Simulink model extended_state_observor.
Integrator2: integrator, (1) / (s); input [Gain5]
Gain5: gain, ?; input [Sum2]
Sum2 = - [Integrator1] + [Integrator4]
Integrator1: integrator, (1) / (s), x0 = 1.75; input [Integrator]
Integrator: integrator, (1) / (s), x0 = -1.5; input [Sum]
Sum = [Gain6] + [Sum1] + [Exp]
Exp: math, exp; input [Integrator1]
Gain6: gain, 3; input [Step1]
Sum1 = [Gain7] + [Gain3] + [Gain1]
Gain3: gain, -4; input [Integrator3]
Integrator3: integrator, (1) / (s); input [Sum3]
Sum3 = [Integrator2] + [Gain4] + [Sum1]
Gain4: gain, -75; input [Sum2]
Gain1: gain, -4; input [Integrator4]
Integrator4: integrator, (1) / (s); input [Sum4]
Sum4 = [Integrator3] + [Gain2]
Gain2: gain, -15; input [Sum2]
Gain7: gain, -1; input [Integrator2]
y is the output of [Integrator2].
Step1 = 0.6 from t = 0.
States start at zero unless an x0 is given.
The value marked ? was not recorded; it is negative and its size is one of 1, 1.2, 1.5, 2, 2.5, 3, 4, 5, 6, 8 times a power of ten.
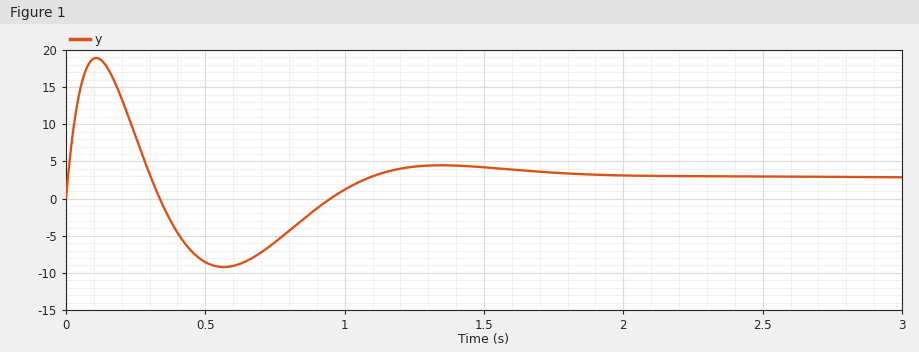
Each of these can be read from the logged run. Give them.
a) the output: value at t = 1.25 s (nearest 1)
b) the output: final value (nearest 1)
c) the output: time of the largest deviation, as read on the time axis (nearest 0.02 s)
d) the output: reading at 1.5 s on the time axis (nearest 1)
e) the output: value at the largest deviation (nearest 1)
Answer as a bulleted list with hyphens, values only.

- 4
- 3
- 0.10 s
- 4
- 19
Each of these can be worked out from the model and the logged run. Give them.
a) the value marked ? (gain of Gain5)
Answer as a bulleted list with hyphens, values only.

- -250
